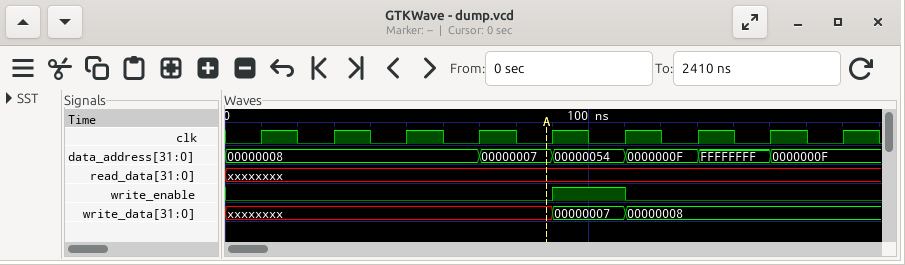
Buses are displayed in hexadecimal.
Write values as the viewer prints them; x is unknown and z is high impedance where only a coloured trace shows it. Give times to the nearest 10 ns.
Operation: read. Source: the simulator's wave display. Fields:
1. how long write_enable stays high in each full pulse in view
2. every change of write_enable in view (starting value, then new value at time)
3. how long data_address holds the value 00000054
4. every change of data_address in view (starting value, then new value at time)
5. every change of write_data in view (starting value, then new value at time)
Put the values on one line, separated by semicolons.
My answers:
20 ns; 0, 1 at 90 ns, 0 at 110 ns; 20 ns; 00000008, 00000007 at 70 ns, 00000054 at 90 ns, 0000000F at 110 ns, FFFFFFFF at 130 ns, 0000000F at 150 ns; xxxxxxxx, 00000007 at 90 ns, 00000008 at 110 ns
